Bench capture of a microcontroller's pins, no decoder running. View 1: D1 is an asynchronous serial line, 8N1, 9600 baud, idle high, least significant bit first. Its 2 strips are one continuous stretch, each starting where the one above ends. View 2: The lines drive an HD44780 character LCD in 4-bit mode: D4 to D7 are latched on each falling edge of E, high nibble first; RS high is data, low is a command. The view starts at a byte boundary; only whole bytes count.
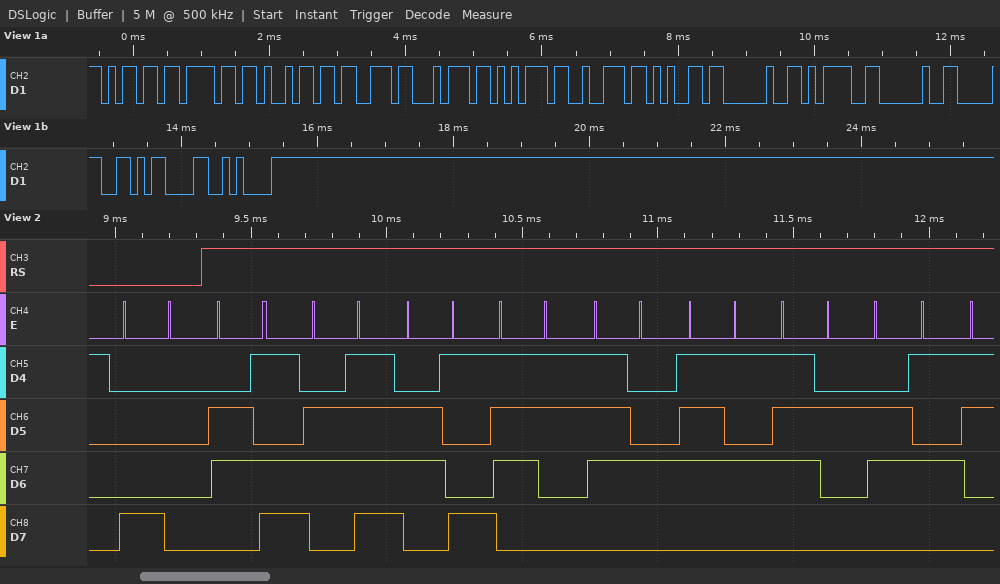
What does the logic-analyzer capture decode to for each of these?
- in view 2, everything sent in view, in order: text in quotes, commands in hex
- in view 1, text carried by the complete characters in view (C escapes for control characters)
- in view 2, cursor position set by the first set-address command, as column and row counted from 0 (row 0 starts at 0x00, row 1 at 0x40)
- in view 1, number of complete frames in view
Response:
0x80 "moisture"
"moisture = 0\r\n"
column 0, row 0
14
